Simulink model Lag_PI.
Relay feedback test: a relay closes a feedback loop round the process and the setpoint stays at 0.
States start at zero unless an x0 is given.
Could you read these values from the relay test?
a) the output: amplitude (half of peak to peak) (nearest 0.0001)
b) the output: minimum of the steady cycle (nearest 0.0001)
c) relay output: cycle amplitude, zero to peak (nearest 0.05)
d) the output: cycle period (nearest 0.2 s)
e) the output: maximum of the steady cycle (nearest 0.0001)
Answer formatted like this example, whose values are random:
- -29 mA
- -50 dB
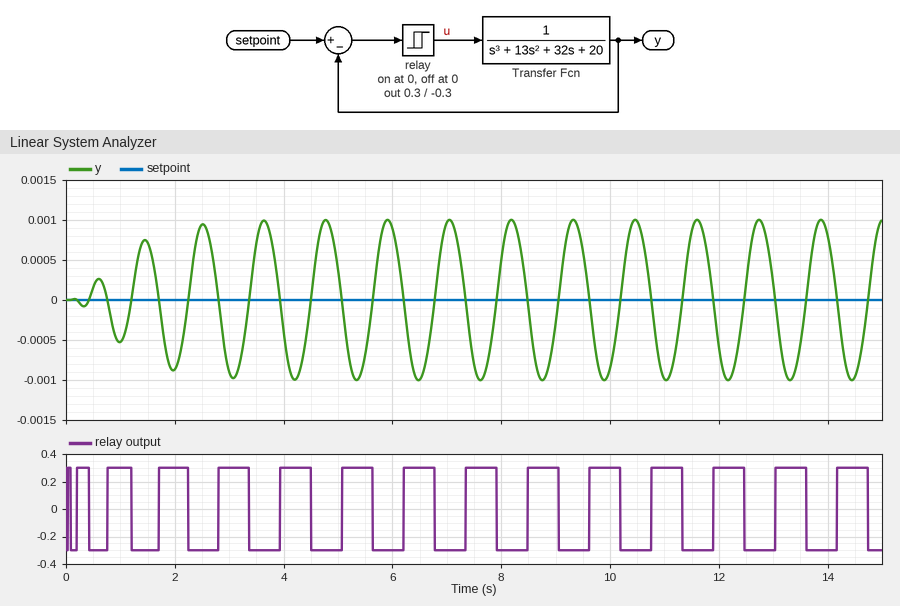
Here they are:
- 0.0010
- -0.0010
- 0.30
- 1.2 s
- 0.0010
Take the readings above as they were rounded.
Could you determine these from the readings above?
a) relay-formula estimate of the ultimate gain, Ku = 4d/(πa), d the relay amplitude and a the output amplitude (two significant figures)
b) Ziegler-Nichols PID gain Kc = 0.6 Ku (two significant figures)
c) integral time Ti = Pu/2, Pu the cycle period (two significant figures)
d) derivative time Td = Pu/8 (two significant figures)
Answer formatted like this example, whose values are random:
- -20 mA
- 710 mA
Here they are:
- 380
- 230
- 0.60 s
- 0.15 s
